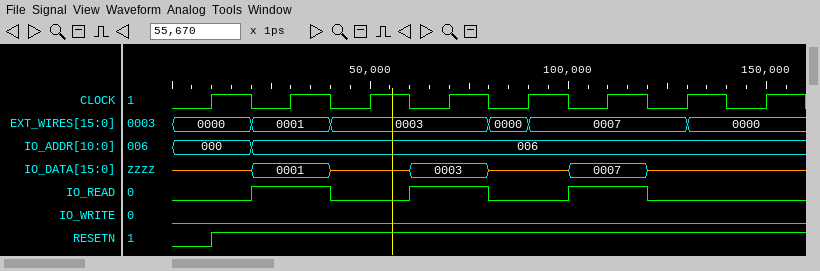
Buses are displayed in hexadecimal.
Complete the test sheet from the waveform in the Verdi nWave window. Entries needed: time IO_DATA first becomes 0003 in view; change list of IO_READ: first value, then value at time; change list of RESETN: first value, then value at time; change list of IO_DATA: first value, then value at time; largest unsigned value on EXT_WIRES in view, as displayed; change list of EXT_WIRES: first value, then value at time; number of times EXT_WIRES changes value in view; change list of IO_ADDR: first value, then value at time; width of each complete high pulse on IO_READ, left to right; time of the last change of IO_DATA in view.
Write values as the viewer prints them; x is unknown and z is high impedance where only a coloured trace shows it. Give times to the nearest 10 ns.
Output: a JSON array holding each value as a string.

["60 ns", "0, 1 at 20 ns, 0 at 40 ns, 1 at 60 ns, 0 at 80 ns, 1 at 100 ns, 0 at 120 ns", "0, 1 at 10 ns", "z, 0001 at 20 ns, z at 40 ns, 0003 at 60 ns, z at 80 ns, 0007 at 100 ns, z at 120 ns", "0007", "0000, 0001 at 20 ns, 0003 at 40 ns, 0000 at 80 ns, 0007 at 90 ns, 0000 at 130 ns", "5", "000, 006 at 20 ns", "20 ns, 20 ns, 20 ns", "120 ns"]
